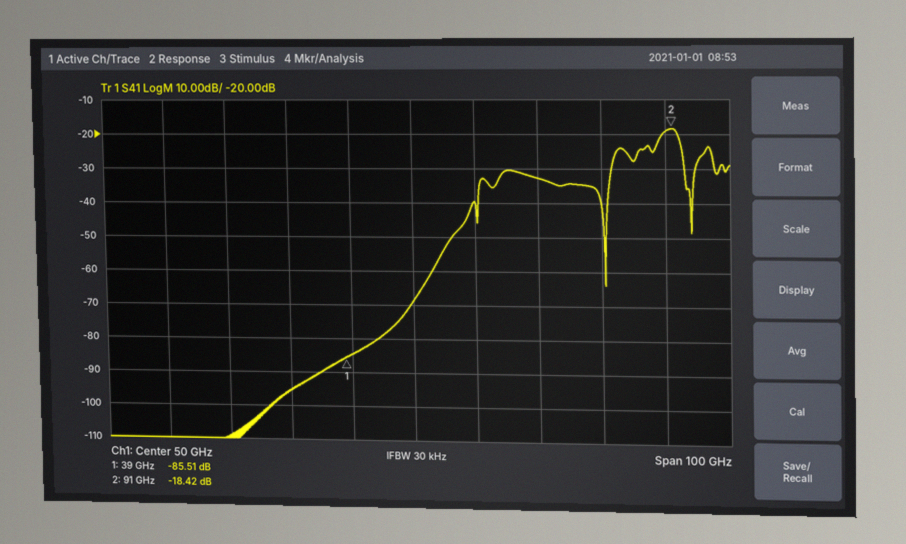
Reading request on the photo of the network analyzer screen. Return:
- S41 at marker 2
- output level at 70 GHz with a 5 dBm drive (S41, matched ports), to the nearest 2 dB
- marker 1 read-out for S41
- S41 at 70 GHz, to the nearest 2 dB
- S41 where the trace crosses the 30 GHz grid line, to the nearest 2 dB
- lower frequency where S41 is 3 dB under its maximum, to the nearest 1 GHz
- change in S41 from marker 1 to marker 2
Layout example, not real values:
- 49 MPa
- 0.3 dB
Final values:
- -18.42 dB
- -28 dBm
- -85.51 dB
- -32 dB
- -96 dB
- 89 GHz
- 67.09 dB
